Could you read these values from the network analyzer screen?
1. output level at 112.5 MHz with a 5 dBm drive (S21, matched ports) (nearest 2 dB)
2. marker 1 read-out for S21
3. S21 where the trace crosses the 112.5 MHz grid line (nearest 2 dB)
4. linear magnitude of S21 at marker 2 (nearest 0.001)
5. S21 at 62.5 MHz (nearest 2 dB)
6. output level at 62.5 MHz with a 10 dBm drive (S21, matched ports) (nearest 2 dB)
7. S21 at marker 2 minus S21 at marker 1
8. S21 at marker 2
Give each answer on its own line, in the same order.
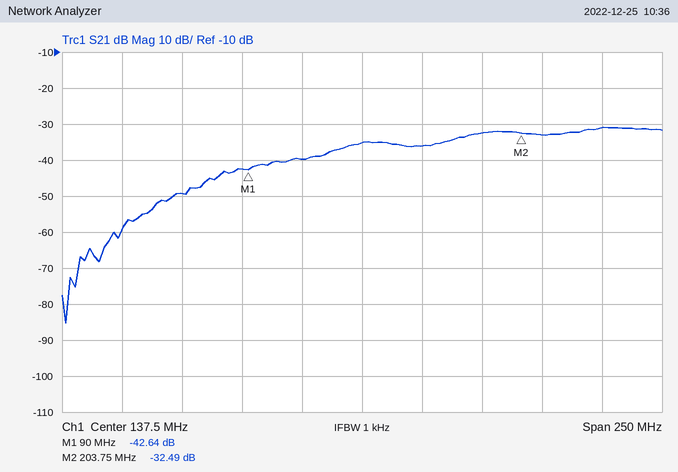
-34 dBm
-42.64 dB
-40 dB
0.024
-50 dB
-40 dBm
10.15 dB
-32.49 dB
